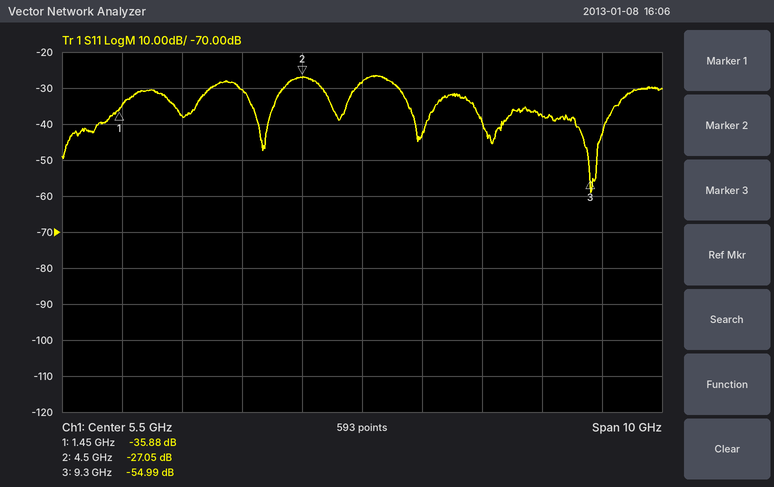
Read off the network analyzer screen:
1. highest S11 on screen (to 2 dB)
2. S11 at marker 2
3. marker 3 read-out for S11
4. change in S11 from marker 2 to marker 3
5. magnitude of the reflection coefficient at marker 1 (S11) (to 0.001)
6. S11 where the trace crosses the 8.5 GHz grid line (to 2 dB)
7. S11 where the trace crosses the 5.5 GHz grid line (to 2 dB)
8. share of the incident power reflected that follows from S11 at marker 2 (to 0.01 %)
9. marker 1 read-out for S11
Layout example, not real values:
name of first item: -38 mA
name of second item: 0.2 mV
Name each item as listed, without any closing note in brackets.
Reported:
highest S11 on screen: -26 dB
S11 at marker 2: -27.05 dB
marker 3 read-out for S11: -54.99 dB
change in S11 from marker 2 to marker 3: -27.94 dB
magnitude of the reflection coefficient at marker 1 (S11): 0.016
S11 where the trace crosses the 8.5 GHz grid line: -38 dB
S11 where the trace crosses the 5.5 GHz grid line: -28 dB
share of the incident power reflected that follows from S11 at marker 2: 0.20 %
marker 1 read-out for S11: -35.88 dB
